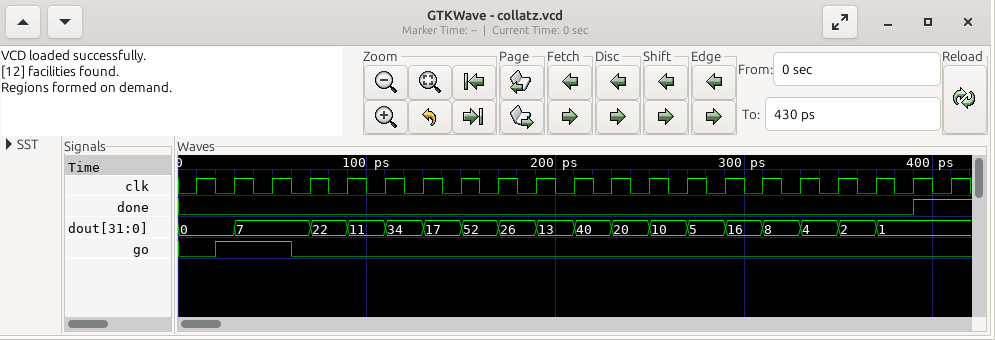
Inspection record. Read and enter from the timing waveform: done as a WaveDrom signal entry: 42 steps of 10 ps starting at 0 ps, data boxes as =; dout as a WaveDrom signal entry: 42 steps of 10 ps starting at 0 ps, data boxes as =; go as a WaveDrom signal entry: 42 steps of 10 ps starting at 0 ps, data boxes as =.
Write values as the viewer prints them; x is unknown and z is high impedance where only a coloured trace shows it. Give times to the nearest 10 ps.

{name: 'done', wave: '0......................................1..'}
{name: 'dout', wave: '=..=...=.=.=.=.=.=.=.=.=.=.=.=.=.=.=.=....', data: '0 7 22 11 34 17 52 26 13 40 20 10 5 16 8 4 2 1'}
{name: 'go', wave: '0.1...0...................................'}
